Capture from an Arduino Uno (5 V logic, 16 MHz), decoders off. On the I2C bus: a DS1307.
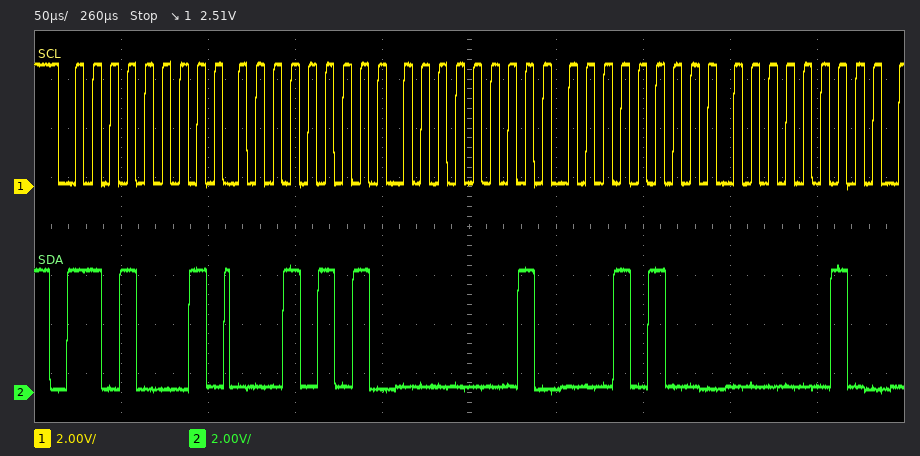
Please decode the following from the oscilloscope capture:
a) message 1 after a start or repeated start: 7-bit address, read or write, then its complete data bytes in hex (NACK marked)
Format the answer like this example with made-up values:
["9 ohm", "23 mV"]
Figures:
["0x68 read: 15 01 14 02"]
